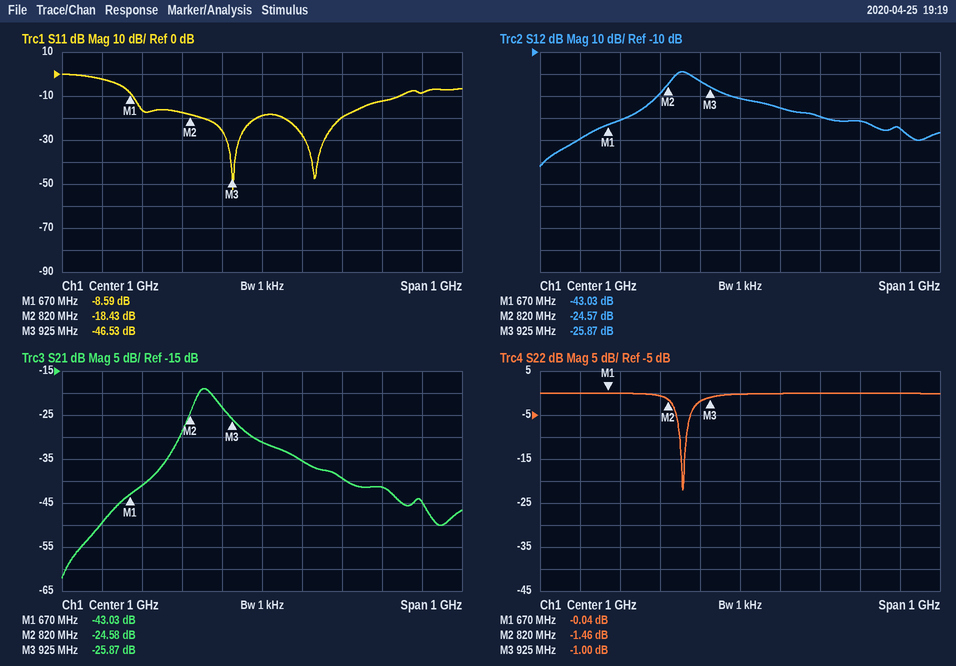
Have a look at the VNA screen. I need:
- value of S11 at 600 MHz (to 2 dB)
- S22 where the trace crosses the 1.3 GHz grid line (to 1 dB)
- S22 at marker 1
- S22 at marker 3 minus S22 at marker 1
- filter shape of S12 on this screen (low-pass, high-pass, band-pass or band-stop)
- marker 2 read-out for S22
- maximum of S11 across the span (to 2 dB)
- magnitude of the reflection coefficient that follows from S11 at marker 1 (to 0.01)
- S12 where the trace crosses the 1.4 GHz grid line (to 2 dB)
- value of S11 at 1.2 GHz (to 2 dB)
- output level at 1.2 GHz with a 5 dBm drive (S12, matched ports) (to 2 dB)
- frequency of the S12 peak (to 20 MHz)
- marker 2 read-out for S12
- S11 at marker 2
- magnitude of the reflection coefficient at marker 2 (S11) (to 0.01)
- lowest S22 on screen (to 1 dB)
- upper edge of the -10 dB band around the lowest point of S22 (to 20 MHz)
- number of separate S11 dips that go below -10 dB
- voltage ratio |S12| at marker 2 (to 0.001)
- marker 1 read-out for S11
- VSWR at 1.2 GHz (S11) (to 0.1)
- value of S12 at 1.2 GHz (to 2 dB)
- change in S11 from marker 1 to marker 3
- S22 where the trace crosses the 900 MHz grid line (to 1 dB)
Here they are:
-2 dB
0 dB
-0.04 dB
-0.96 dB
band-pass
-1.46 dB
0 dB
0.37
-44 dB
-20 dB
-34 dBm
860 MHz
-24.57 dB
-18.43 dB
0.12
-22 dB
860 MHz
2
0.059
-8.59 dB
1.2
-40 dB
-37.94 dB
-2 dB
